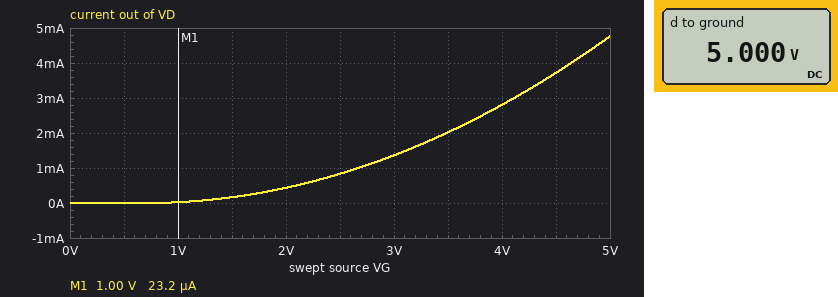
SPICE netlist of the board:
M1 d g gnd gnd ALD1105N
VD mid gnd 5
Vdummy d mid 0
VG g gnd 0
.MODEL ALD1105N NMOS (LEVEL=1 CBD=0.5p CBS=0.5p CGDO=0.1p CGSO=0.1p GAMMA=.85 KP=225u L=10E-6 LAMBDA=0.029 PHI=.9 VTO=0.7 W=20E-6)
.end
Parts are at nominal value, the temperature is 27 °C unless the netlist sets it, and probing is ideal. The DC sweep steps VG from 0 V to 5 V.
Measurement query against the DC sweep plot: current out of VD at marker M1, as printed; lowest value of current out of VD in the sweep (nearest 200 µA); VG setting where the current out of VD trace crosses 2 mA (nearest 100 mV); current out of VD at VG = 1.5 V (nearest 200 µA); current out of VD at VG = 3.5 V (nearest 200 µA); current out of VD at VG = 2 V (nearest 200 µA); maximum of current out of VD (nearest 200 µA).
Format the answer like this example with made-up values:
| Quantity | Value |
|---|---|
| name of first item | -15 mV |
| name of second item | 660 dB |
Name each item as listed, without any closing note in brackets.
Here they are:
| Quantity | Value |
|---|---|
| current out of VD at marker M1, as printed | 23.2 µA |
| lowest value of current out of VD in the sweep | 0 A |
| VG setting where the current out of VD trace crosses 2 mA | 3.5 V |
| current out of VD at VG = 1.5 V | 200 µA |
| current out of VD at VG = 3.5 V | 2.0 mA |
| current out of VD at VG = 2 V | 400 µA |
| maximum of current out of VD | 4.8 mA |
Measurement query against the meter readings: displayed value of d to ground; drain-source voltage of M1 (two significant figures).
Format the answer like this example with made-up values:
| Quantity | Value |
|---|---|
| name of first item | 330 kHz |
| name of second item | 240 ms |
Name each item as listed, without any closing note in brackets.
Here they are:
| Quantity | Value |
|---|---|
| displayed value of d to ground | 5.000 V |
| drain-source voltage of M1 | 5.0 V |
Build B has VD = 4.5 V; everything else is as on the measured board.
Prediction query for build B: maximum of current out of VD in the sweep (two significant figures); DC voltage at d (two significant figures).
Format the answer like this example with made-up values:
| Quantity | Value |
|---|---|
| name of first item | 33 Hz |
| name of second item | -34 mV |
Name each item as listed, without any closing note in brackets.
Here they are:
| Quantity | Value |
|---|---|
| maximum of current out of VD in the sweep | 4.7 mA |
| DC voltage at d | 4.5 V |
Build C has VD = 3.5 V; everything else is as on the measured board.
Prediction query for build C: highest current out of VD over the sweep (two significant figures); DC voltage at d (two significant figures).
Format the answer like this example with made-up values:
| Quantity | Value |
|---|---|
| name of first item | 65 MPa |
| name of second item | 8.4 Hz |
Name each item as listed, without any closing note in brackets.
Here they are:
| Quantity | Value |
|---|---|
| highest current out of VD over the sweep | 4.4 mA |
| DC voltage at d | 3.5 V |
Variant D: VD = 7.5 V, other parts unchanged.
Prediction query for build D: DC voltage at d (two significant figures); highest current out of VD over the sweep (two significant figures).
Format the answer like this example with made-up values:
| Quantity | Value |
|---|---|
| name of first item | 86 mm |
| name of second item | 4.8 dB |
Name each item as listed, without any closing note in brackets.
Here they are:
| Quantity | Value |
|---|---|
| DC voltage at d | 7.5 V |
| highest current out of VD over the sweep | 5.1 mA |
